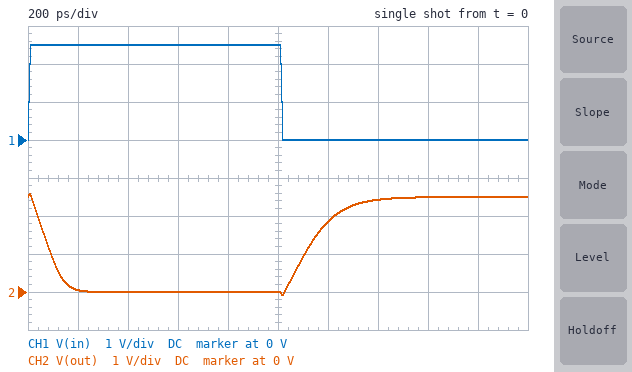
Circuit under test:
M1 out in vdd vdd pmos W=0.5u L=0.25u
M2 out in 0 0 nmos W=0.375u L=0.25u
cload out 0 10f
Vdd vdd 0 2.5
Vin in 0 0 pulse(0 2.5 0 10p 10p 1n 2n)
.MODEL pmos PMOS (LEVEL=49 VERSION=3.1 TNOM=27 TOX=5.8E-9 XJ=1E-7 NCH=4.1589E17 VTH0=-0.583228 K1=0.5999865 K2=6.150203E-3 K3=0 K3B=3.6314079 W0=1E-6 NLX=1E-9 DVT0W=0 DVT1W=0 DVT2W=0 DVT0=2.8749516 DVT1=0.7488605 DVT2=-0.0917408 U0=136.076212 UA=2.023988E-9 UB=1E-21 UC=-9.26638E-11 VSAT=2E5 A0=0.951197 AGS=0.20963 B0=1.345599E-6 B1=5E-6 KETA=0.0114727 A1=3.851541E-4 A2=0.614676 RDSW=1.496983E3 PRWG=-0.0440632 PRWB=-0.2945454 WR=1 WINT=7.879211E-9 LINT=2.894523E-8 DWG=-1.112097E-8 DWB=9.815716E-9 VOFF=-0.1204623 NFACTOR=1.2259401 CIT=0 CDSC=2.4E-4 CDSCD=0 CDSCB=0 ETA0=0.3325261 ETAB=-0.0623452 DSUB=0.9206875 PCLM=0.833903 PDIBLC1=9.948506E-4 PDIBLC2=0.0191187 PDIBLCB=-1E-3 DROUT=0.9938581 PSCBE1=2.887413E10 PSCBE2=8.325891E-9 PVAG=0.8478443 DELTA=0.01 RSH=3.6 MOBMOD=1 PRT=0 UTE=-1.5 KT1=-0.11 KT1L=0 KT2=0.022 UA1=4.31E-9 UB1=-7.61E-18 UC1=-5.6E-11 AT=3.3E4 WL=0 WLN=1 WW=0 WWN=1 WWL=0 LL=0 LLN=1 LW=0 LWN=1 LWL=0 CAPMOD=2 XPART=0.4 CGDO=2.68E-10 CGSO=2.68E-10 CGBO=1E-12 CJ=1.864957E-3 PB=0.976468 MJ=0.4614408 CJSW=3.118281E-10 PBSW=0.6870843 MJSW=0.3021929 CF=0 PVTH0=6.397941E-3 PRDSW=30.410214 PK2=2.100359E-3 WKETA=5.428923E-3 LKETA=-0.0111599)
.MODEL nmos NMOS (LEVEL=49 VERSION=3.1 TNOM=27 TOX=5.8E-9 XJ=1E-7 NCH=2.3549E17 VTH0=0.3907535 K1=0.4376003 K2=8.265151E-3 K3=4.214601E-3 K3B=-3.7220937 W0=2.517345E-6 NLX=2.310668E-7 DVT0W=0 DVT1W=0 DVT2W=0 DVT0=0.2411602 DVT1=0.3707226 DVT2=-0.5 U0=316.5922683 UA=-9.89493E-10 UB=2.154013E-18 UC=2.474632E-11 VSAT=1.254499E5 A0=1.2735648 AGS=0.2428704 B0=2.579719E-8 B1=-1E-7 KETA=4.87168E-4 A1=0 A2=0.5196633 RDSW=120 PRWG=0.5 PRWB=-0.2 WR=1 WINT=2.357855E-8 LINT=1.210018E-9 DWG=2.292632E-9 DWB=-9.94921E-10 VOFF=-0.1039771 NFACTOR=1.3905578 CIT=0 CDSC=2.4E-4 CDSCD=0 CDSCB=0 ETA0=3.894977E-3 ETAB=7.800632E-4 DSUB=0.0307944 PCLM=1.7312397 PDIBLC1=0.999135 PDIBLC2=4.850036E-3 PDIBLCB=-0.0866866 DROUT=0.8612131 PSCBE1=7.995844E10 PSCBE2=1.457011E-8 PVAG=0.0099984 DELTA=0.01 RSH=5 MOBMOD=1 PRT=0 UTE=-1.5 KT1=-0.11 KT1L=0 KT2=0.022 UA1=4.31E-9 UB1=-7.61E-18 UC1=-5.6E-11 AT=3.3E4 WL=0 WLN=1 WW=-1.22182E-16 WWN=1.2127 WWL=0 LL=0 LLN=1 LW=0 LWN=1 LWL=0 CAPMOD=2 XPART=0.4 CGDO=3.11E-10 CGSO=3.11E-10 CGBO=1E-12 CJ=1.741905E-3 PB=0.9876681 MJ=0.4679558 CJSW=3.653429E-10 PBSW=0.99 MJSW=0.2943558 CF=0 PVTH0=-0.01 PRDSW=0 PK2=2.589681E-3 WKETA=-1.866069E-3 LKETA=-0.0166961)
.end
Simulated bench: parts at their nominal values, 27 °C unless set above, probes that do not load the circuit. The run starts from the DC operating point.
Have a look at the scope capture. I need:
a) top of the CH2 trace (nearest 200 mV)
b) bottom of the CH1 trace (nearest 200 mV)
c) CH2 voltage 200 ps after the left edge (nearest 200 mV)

2.6 V
0 V
0 V
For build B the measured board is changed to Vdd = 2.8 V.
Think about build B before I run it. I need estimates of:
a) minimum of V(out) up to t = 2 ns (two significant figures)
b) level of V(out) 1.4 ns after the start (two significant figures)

-77 mV
2.7 V
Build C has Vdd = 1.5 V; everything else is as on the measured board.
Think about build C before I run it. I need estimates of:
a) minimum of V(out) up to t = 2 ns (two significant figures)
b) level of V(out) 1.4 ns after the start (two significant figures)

-110 mV
1.3 V
